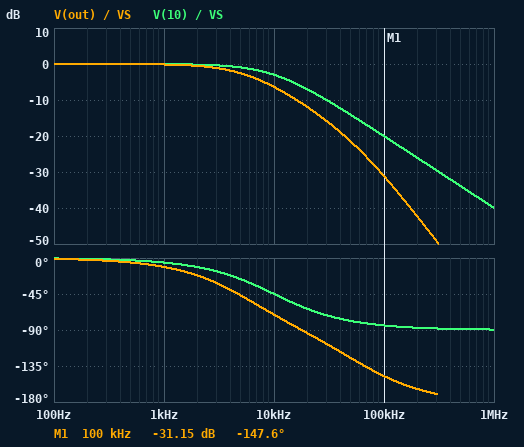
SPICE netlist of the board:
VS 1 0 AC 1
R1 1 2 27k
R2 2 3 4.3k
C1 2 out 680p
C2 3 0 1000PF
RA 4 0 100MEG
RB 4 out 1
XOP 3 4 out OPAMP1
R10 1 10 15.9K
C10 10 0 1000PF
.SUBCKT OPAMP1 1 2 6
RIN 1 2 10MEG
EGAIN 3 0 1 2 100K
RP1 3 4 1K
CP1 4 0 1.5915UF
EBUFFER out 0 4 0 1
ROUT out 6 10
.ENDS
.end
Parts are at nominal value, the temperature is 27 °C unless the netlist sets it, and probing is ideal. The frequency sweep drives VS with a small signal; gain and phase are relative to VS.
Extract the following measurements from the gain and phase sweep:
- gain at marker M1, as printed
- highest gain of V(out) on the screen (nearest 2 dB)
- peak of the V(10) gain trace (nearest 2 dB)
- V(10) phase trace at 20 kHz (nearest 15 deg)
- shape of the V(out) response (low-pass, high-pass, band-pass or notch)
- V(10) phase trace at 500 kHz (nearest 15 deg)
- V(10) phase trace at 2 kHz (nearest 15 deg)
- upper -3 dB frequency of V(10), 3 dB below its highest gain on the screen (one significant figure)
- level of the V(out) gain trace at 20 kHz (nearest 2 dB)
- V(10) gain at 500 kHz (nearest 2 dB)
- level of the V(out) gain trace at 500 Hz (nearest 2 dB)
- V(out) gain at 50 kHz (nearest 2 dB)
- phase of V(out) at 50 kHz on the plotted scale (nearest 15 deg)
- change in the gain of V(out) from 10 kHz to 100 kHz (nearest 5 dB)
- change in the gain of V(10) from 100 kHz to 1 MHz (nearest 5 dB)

-31.15 dB
0 dB
0 dB
-60 deg
low-pass
-90 deg
-15 deg
10 kHz
-12 dB
-34 dB
0 dB
-22 dB
-120 deg
-25 dB
-20 dB
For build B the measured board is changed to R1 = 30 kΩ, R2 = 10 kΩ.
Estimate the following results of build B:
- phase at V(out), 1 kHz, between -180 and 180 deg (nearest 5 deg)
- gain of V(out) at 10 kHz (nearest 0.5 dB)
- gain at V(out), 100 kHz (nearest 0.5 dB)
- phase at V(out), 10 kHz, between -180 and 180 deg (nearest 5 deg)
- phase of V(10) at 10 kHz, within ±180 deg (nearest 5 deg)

-15 deg
-8.0 dB
-38.5 dB
-85 deg
-45 deg
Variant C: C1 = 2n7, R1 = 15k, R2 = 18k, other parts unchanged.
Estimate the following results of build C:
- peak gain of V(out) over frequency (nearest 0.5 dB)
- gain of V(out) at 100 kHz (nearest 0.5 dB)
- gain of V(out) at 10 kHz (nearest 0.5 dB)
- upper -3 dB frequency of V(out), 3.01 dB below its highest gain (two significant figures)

0.5 dB
-49.0 dB
-9.0 dB
6.5 kHz
